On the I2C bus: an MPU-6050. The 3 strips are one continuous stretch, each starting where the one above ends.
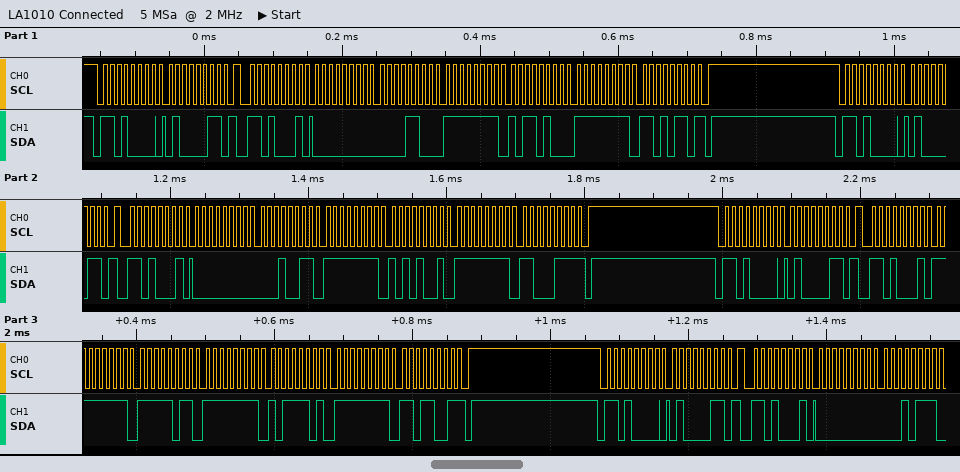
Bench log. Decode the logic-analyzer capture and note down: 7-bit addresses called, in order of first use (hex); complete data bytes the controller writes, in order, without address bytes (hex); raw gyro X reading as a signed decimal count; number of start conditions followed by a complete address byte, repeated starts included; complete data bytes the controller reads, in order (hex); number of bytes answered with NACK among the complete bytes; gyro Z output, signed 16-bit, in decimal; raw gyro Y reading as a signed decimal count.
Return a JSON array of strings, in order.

["0x68", "43 43 43 43", "12", "8", "00 0C FF B4 FF D6 00 13 FF A9 FF C7 FF FB FF BD FF D9 00 17", "3", "-42", "-76"]
